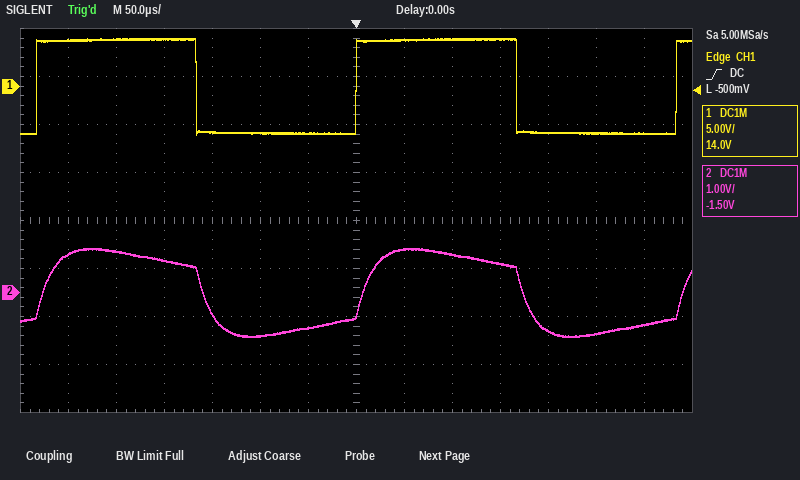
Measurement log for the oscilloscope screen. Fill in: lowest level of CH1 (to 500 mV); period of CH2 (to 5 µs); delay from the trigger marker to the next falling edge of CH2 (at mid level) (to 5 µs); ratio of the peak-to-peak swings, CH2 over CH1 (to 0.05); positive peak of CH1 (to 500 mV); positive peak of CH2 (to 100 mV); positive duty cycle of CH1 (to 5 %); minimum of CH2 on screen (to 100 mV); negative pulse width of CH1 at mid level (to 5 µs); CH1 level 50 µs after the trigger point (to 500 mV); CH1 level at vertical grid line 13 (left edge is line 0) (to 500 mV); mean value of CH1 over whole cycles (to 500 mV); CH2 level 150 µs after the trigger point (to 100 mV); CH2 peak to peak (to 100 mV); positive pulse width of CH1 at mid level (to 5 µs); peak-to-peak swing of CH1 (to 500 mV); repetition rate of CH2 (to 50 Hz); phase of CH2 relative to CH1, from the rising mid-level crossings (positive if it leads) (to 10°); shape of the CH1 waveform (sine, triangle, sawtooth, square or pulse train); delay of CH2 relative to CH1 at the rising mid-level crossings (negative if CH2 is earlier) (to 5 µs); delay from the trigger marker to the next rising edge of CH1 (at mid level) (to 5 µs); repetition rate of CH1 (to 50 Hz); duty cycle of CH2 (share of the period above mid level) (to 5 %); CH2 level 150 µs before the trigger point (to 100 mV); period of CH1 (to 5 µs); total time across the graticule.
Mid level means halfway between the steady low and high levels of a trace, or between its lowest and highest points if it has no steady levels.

-5.0 V
335 µs
175 µs
0.20
5.0 V
900 mV
50 %
-900 mV
165 µs
5.0 V
-5.0 V
0.0 V
600 mV
1.8 V
165 µs
10.0 V
3.00 kHz
-10°
square
+5 µs
335 µs
3.00 kHz
50 %
-400 mV
335 µs
700 µs
